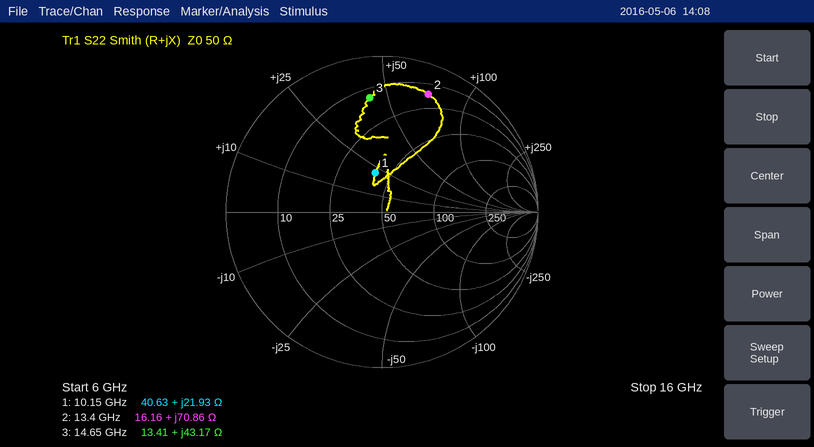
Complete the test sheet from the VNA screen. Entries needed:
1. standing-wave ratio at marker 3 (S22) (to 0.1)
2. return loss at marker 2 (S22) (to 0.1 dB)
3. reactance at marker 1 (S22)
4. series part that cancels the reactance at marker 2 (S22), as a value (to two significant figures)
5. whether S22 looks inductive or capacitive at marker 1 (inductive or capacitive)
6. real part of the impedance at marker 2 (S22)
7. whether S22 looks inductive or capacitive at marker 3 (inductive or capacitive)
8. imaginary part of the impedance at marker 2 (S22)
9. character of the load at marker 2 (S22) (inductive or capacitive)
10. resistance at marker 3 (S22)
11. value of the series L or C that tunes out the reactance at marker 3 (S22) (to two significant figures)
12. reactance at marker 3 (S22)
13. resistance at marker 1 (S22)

6.6
1.8 dB
+21.93 Ω
170 fF
inductive
16.16 Ω
inductive
+70.86 Ω
inductive
13.41 Ω
250 fF
+43.17 Ω
40.63 Ω
